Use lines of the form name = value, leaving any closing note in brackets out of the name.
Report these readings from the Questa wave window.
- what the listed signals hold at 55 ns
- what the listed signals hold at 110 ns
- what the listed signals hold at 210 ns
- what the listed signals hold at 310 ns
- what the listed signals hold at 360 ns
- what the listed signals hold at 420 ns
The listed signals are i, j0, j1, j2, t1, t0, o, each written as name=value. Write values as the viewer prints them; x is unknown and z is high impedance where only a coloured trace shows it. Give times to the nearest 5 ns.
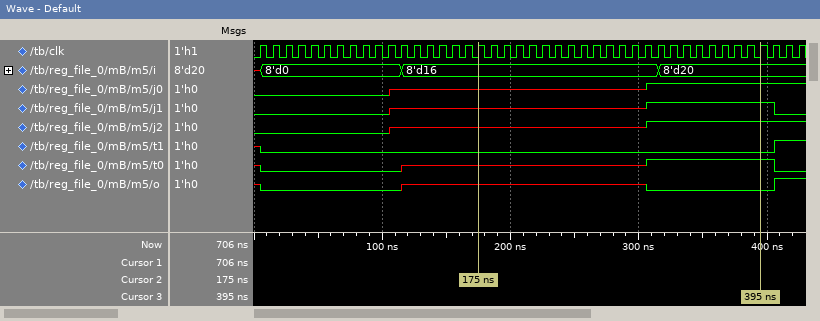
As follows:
what the listed signals hold at 55 ns = i=8'd0, j0=0, j1=0, j2=0, t1=0, t0=0, o=0
what the listed signals hold at 110 ns = i=8'd0, j0=x, j1=x, j2=x, t1=0, t0=0, o=0
what the listed signals hold at 210 ns = i=8'd16, j0=x, j1=x, j2=x, t1=0, t0=x, o=x
what the listed signals hold at 310 ns = i=8'd16, j0=1, j1=1, j2=1, t1=0, t0=1, o=0
what the listed signals hold at 360 ns = i=8'd20, j0=1, j1=1, j2=1, t1=0, t0=1, o=0
what the listed signals hold at 420 ns = i=8'd20, j0=1, j1=0, j2=1, t1=1, t0=0, o=1
